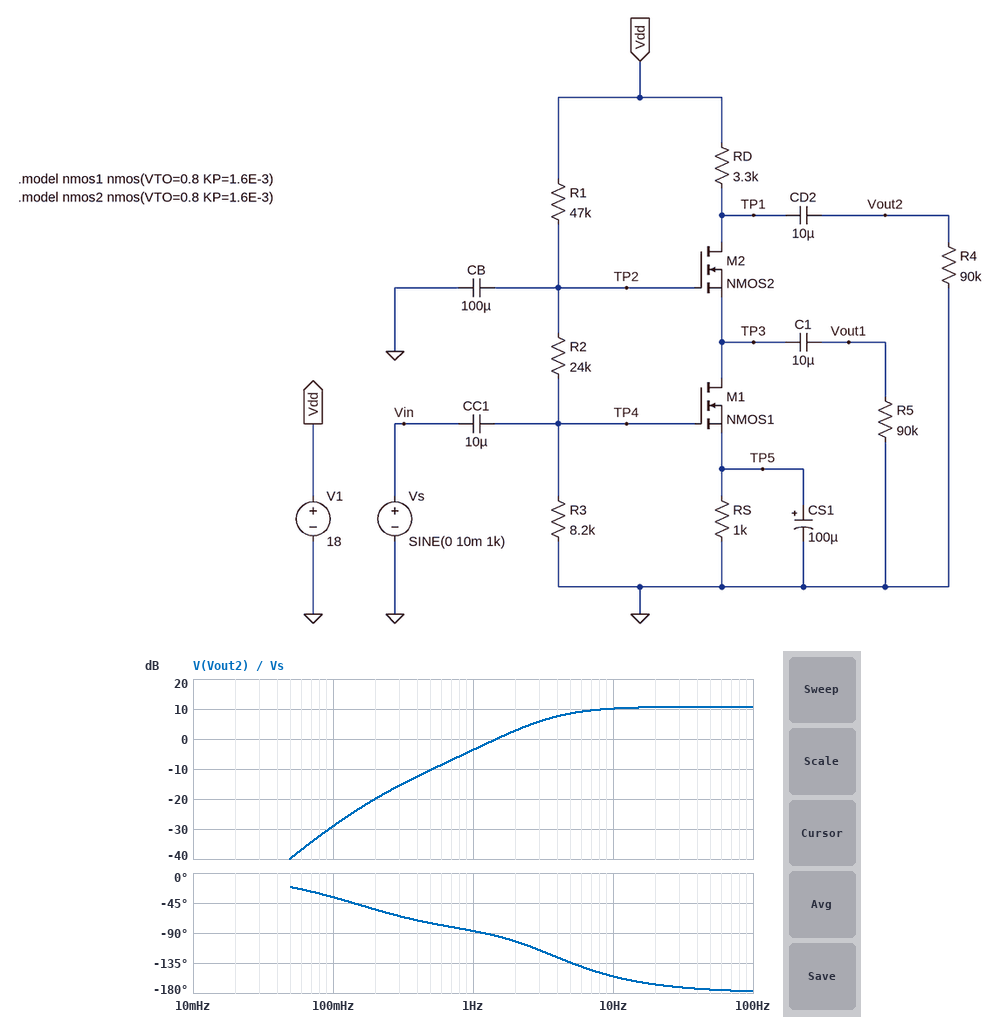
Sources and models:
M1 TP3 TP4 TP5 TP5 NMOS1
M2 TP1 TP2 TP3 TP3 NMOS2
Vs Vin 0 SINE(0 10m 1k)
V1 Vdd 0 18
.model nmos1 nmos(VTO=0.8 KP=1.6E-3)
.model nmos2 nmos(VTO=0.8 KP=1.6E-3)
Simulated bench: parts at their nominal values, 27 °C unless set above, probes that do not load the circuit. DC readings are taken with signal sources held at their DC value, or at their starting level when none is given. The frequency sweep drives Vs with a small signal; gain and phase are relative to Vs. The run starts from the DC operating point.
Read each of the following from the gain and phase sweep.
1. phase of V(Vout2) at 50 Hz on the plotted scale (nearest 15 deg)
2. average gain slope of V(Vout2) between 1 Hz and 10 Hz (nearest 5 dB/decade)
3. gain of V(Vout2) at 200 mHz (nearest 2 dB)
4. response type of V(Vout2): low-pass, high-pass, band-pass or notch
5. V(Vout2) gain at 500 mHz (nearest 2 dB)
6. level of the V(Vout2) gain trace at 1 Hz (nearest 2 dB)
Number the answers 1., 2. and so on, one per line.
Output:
1. -180 deg
2. 15 dB/decade
3. -20 dB
4. high-pass
5. -10 dB
6. -4 dB
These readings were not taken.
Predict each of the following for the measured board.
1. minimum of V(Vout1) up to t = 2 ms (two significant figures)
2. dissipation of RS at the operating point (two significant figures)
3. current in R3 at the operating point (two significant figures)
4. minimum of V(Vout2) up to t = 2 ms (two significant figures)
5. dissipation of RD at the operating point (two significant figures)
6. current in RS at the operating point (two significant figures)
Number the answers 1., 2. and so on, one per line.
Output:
1. -9.9 mV
2. 140 µW
3. 230 µA
4. -35 mV
5. 470 µW
6. 380 µA
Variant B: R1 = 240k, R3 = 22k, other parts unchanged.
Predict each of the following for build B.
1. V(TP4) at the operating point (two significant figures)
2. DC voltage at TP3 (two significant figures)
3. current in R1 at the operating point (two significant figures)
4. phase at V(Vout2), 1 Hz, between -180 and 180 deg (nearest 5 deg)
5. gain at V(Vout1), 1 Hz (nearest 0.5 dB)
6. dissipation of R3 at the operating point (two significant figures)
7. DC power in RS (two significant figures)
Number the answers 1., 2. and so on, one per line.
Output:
1. 1.4 V
2. 1.7 V
3. 63 µA
4. -105 deg
5. -8.5 dB
6. 87 µW
7. 23 µW
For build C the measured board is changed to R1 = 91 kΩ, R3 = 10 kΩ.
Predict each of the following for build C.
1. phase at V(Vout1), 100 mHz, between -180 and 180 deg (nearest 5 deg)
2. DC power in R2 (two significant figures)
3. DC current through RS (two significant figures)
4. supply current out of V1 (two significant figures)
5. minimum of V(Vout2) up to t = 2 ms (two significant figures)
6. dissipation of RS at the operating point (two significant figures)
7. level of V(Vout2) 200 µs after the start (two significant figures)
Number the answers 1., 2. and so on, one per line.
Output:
1. 20 deg
2. 500 µW
3. 170 µA
4. 320 µA
5. -24 mV
6. 30 µW
7. -22 mV
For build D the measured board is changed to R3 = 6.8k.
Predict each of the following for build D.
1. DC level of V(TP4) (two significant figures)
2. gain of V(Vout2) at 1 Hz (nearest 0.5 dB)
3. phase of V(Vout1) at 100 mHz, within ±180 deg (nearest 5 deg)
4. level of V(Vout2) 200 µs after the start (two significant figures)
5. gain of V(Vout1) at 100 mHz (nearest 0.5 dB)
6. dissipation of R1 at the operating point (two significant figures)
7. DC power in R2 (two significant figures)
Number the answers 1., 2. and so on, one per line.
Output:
1. 1.6 V
2. -6.0 dB
3. 25 deg
4. -26 mV
5. -43.0 dB
6. 2.5 mW
7. 1.3 mW
